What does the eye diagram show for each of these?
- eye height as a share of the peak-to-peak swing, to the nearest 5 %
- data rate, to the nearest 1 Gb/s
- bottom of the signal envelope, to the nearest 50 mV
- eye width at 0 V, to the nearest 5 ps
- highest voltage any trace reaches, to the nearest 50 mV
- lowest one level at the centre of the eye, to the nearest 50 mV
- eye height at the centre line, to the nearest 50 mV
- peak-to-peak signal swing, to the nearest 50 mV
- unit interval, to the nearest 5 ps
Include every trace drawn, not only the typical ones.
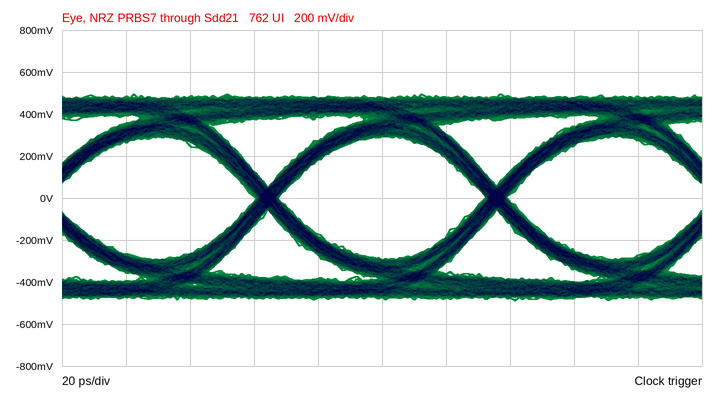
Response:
60 %
14 Gb/s
-500 mV
65 ps
500 mV
300 mV
600 mV
1.00 V
70 ps
